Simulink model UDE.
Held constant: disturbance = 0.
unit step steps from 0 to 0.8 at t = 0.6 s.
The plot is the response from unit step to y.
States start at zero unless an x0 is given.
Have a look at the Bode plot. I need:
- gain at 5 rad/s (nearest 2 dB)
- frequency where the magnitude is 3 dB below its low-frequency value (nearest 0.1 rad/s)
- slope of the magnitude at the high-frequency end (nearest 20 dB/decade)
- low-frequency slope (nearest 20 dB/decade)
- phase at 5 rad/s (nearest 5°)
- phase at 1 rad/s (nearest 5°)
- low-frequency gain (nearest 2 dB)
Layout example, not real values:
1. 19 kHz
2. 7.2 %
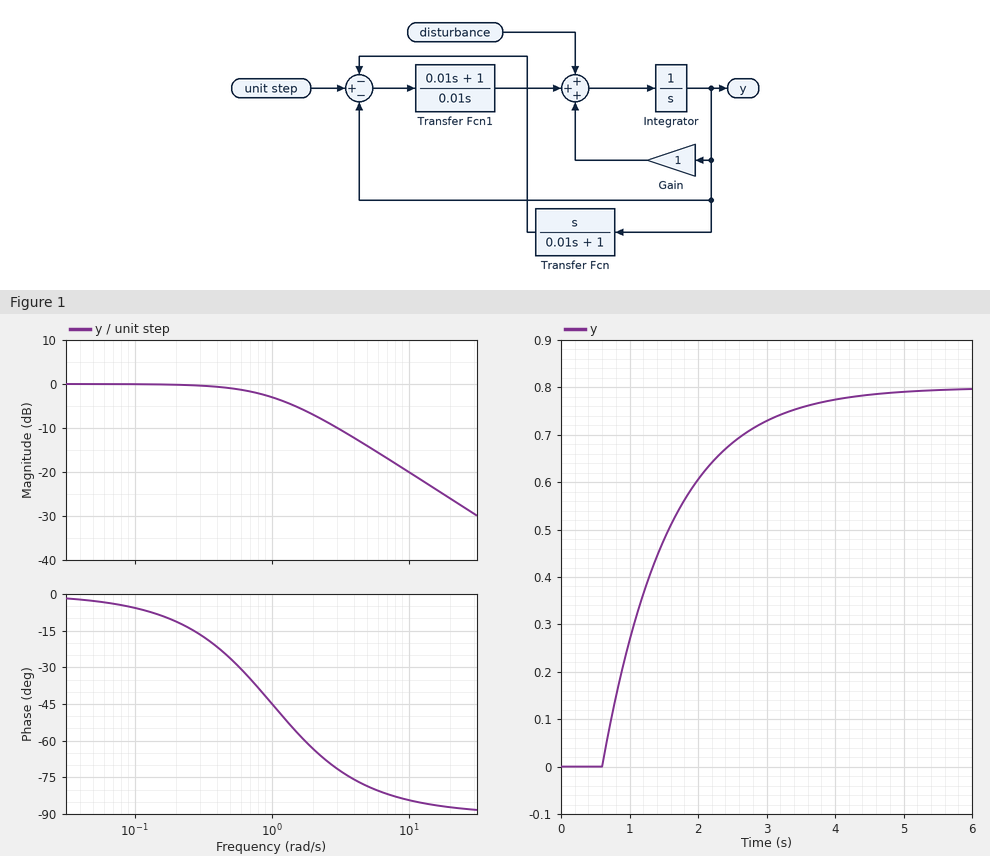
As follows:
1. -14 dB
2. 1.0 rad/s
3. -20 dB/decade
4. 0 dB/decade
5. -80°
6. -45°
7. 0 dB
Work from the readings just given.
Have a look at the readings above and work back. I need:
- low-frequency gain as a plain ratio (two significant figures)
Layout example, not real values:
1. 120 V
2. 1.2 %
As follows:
1. 1.0
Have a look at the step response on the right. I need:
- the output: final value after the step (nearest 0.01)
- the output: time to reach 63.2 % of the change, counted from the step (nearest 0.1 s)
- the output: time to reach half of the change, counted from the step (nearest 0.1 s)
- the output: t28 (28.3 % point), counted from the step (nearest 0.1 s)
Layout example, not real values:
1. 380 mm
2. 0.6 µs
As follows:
1. 0.80
2. 1.0 s
3. 0.7 s
4. 0.3 s
